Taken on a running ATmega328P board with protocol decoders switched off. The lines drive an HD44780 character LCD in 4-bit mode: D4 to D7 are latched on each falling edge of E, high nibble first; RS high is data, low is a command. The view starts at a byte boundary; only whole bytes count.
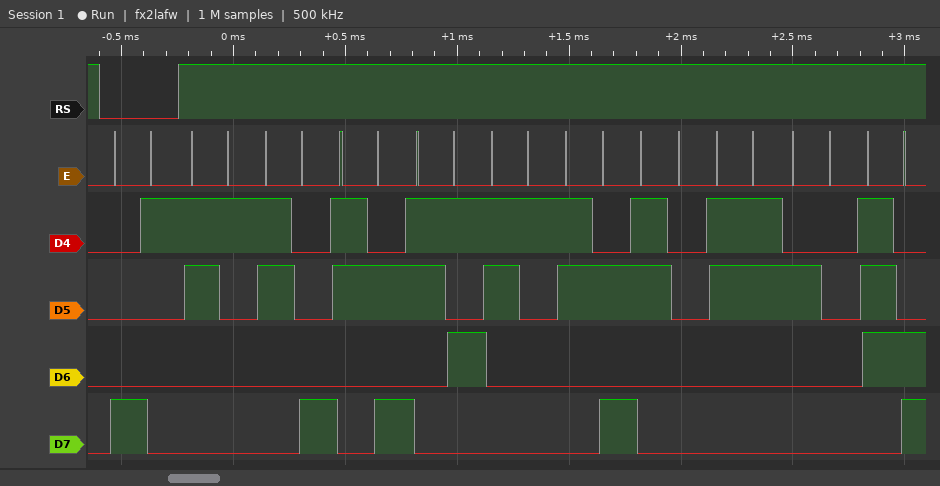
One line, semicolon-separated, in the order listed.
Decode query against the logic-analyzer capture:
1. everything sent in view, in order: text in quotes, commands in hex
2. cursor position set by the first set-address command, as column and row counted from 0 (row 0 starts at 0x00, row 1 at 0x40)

0x81 "18:51:03 |"; column 1, row 0
